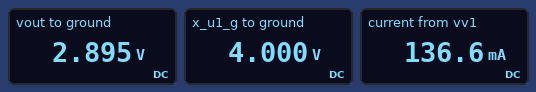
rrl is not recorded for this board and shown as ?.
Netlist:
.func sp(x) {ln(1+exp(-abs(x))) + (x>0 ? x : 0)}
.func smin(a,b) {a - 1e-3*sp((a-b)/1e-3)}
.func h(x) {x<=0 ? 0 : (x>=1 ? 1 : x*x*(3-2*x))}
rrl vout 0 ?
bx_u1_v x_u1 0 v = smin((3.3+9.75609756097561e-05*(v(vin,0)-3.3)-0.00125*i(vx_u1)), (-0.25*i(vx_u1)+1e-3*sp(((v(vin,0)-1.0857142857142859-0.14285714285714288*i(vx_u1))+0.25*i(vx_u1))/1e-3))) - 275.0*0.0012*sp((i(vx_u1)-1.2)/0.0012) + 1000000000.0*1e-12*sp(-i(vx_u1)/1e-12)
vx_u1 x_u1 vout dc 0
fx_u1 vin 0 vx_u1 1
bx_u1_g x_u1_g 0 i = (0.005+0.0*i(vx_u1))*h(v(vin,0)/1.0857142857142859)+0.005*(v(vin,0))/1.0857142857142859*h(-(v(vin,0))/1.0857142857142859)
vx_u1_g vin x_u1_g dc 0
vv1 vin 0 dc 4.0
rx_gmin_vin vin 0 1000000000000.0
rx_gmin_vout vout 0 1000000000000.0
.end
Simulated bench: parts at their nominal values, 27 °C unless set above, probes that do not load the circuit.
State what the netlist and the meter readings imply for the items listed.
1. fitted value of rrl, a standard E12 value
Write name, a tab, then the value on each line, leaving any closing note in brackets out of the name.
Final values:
fitted value of rrl, a standard E12 value	22 Ω
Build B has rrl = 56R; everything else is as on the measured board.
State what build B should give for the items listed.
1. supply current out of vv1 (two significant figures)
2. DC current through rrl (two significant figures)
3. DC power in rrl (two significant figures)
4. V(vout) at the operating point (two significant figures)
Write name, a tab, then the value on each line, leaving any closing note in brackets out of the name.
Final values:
supply current out of vv1	57 mA
DC current through rrl	52 mA
DC power in rrl	150 mW
V(vout) at the operating point	2.9 V
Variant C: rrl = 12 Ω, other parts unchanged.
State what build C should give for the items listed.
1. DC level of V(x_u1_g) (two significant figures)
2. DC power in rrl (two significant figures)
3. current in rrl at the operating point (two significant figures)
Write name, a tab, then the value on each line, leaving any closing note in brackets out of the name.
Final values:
DC level of V(x_u1_g)	4.0 V
DC power in rrl	690 mW
current in rrl at the operating point	240 mA
